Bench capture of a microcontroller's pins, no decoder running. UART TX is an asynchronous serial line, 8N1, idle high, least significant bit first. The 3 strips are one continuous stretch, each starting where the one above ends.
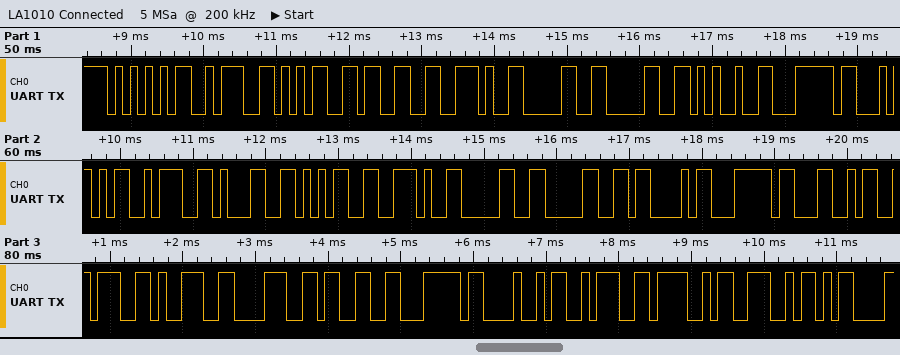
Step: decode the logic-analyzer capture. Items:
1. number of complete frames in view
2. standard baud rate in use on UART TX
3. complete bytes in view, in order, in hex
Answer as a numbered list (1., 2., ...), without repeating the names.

1. 29
2. 9600 baud
3. 55 3A 35 33 2E 30 30 25 7C 54 3A 31 35 2E 30 30 43 7C 4C 3A 39 38 33 7C 48 3A 4F 4E 0D
